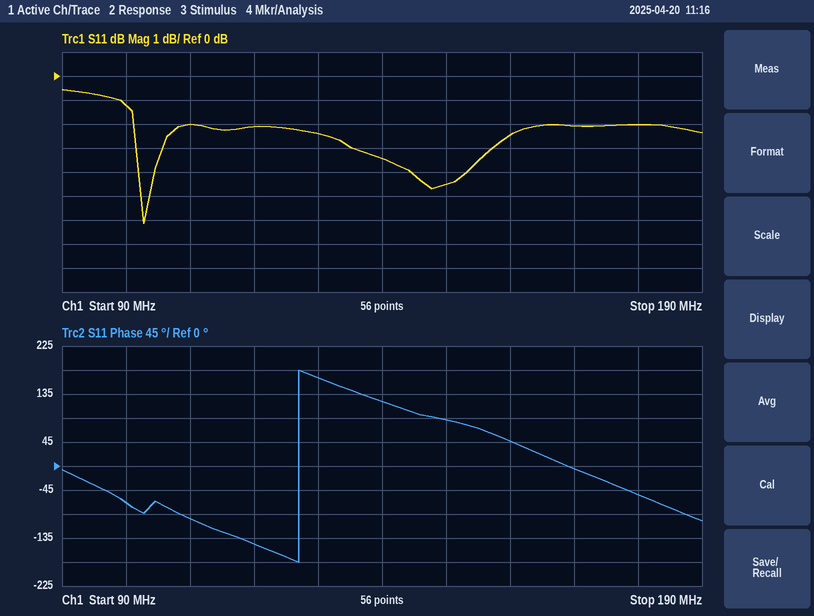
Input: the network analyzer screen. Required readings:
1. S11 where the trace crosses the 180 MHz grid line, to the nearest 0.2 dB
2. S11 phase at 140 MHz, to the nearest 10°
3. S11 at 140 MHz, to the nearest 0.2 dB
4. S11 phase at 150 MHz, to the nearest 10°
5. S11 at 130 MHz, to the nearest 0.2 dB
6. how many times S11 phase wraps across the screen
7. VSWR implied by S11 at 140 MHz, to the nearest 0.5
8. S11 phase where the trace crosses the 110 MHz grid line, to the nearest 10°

-2.0 dB
120°
-3.4 dB
90°
-2.4 dB
1
5.0
-100°
